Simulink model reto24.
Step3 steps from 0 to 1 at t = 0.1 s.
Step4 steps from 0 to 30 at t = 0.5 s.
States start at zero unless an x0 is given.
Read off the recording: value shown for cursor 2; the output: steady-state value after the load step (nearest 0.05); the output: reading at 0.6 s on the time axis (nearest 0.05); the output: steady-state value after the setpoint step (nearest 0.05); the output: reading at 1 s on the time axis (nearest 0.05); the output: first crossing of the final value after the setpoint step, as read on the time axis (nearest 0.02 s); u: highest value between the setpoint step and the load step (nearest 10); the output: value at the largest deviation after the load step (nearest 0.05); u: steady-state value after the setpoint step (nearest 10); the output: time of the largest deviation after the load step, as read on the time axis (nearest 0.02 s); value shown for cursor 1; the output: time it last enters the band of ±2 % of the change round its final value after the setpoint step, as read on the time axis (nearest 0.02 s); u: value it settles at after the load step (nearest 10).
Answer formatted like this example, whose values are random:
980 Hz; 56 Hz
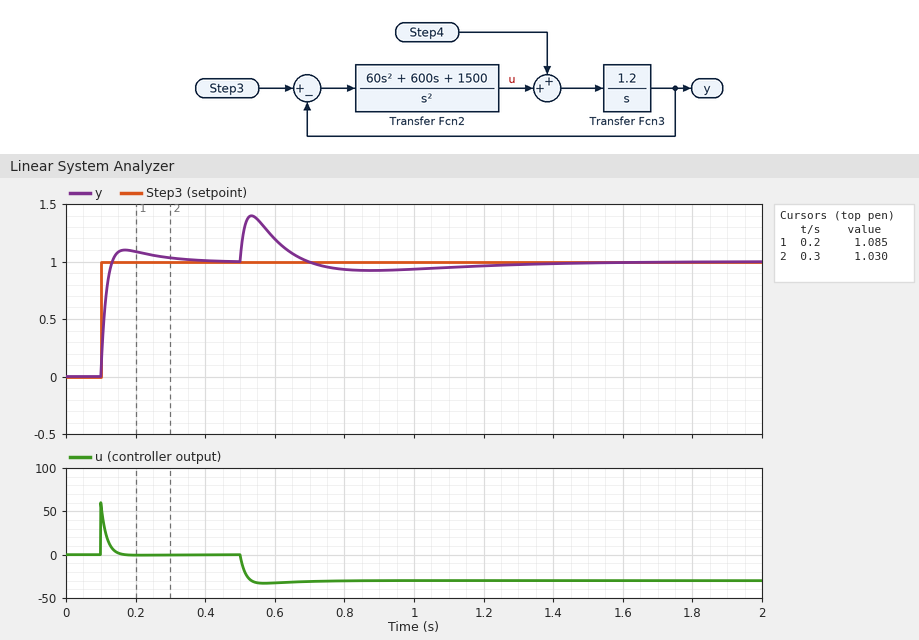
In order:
1.030; 1.00; 1.20; 1.00; 0.95; 0.14 s; 60; 1.40; 0; 0.54 s; 1.085; 0.34 s; -30
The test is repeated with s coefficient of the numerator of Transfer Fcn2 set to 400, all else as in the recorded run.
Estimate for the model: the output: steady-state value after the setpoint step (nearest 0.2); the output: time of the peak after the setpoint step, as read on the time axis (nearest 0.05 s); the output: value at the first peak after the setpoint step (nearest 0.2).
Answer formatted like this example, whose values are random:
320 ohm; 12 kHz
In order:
1.0; 0.20 s; 1.0
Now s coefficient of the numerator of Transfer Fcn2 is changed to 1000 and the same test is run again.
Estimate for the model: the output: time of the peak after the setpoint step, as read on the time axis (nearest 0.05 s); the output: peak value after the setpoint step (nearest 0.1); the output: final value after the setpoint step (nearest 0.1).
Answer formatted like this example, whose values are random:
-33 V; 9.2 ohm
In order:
0.15 s; 1.1; 1.0
